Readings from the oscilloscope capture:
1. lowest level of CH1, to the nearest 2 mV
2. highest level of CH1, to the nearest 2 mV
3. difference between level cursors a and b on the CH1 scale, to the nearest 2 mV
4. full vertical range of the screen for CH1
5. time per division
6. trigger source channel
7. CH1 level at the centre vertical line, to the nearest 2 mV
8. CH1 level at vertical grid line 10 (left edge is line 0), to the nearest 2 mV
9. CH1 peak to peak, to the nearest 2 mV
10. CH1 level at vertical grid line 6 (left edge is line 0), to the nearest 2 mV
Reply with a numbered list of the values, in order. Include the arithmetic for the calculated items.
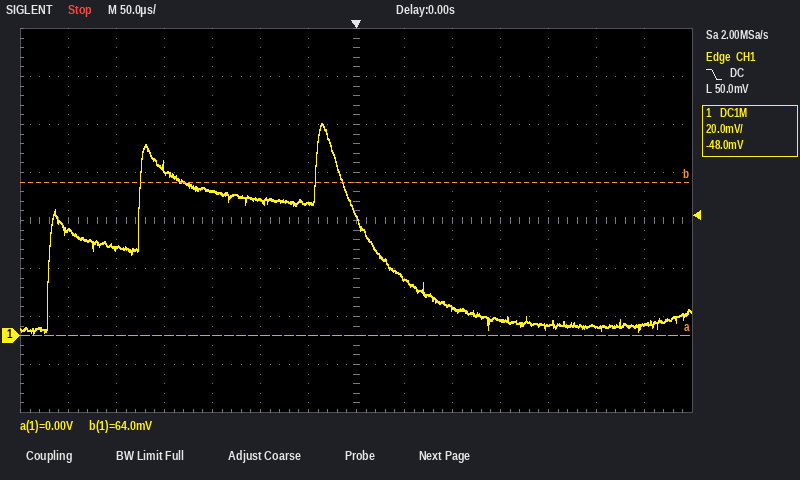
1. 0 mV
2. 88 mV
3. 64 mV
4. 160 mV
5. 50 µs
6. CH1
7. 50 mV
8. 6 mV
9. 88 mV − (0 mV) = 88 mV
10. 56 mV
